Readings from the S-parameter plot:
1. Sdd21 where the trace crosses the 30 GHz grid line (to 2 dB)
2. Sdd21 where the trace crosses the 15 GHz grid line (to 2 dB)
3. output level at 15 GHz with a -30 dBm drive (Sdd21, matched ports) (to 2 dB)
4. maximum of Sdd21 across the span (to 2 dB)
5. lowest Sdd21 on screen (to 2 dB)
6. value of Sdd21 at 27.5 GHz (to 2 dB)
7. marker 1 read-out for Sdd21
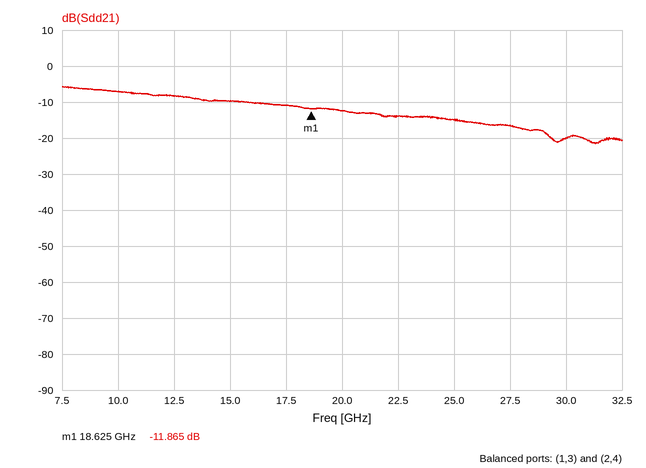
-20 dB
-10 dB
-40 dBm
-6 dB
-22 dB
-16 dB
-11.865 dB
